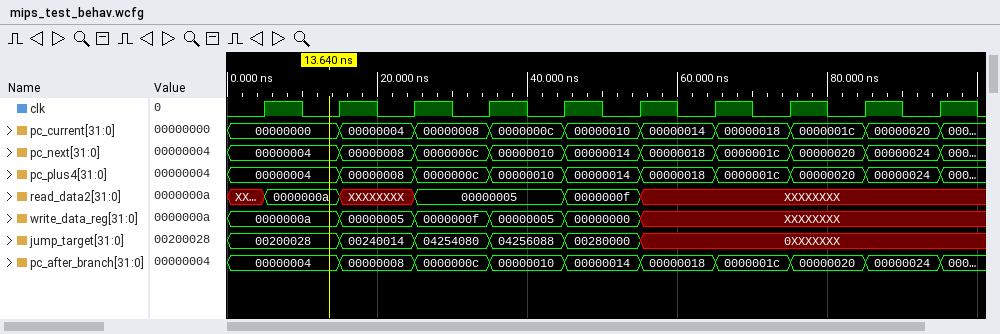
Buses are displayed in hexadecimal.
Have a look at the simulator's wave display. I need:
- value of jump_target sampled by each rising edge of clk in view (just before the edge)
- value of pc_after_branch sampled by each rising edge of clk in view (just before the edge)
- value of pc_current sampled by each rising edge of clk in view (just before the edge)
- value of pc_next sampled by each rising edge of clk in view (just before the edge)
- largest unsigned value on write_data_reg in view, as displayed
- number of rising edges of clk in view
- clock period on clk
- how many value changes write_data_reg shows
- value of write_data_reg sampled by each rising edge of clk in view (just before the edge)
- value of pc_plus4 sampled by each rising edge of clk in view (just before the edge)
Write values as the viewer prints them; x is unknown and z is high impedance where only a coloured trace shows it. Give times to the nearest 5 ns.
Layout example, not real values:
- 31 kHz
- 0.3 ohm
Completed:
- 00200028, 00200028, 00240014, 04254080, 04256088, 00280000, 0XXXXXXX, 0XXXXXXX, 0XXXXXXX, 0XXXXXXX
- 00000004, 00000004, 00000008, 0000000c, 00000010, 00000014, 00000018, 0000001c, 00000020, 00000024
- 00000000, 00000000, 00000004, 00000008, 0000000c, 00000010, 00000014, 00000018, 0000001c, 00000020
- 00000004, 00000004, 00000008, 0000000c, 00000010, 00000014, 00000018, 0000001c, 00000020, 00000024
- 0000000f
- 10
- 10 ns
- 5
- 0000000a, 0000000a, 00000005, 0000000f, 00000005, 00000000, XXXXXXXX, XXXXXXXX, XXXXXXXX, XXXXXXXX
- 00000004, 00000004, 00000008, 0000000c, 00000010, 00000014, 00000018, 0000001c, 00000020, 00000024
